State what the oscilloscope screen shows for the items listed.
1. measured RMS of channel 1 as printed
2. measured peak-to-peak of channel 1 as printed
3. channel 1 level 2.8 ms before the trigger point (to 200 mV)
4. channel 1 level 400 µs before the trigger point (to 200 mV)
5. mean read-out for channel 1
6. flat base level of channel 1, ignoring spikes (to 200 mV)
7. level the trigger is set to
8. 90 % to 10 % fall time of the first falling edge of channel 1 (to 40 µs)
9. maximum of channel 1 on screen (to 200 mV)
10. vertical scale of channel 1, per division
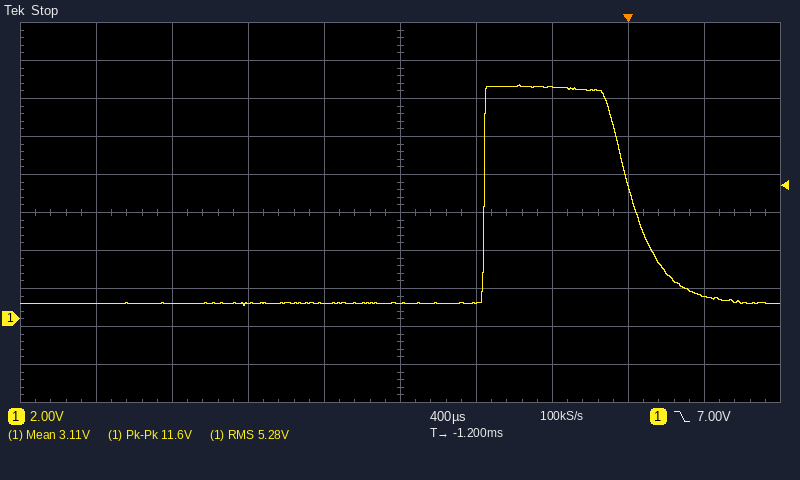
5.28 V
11.6 V
800 mV
12.2 V
3.11 V
800 mV
7.00 V
360 µs
12.4 V
2 V
